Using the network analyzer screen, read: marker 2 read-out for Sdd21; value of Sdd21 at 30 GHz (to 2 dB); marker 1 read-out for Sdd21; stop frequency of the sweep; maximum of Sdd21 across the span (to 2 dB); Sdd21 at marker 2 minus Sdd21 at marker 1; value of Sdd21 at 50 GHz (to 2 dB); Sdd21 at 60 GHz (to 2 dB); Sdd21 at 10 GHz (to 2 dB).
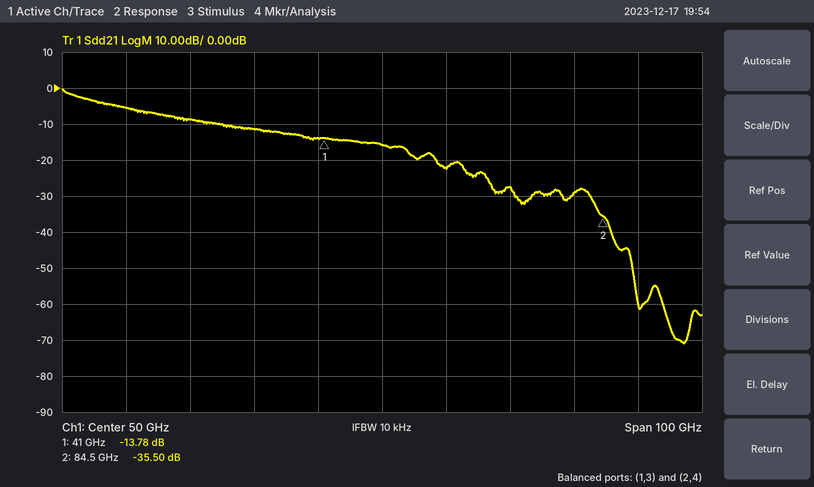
-35.50 dB
-12 dB
-13.78 dB
100 GHz
0 dB
-21.72 dB
-16 dB
-22 dB
-6 dB
